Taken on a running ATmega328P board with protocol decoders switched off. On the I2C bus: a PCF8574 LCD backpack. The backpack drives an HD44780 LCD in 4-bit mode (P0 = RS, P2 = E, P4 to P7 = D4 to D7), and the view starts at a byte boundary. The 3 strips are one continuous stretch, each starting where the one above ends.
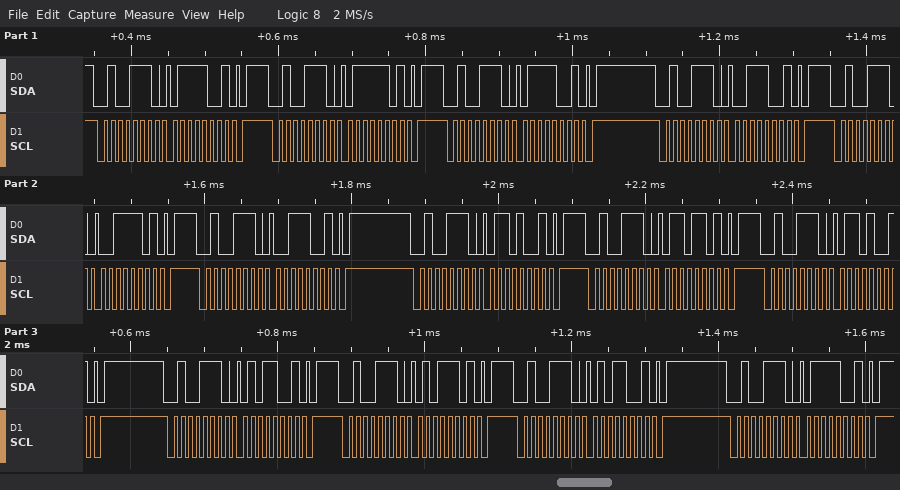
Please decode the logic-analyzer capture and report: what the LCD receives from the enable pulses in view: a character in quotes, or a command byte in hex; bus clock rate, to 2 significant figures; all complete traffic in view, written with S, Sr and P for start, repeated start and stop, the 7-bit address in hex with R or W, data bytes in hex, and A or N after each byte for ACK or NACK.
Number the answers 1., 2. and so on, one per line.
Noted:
1. 's' 'e'
2. 100 kHz
3. S 27W A 79 A P S 27W A 7D A P S 27W A 79 A P S 27W A 39 A P S 27W A 3D A P S 27W A 39 A P S 27W A 69 A P S 27W A 6D A P S 27W A 69 A P S 27W A 59 A P S 27W A 5D A P S 27W A 59 A P S 27W A 79 A P
